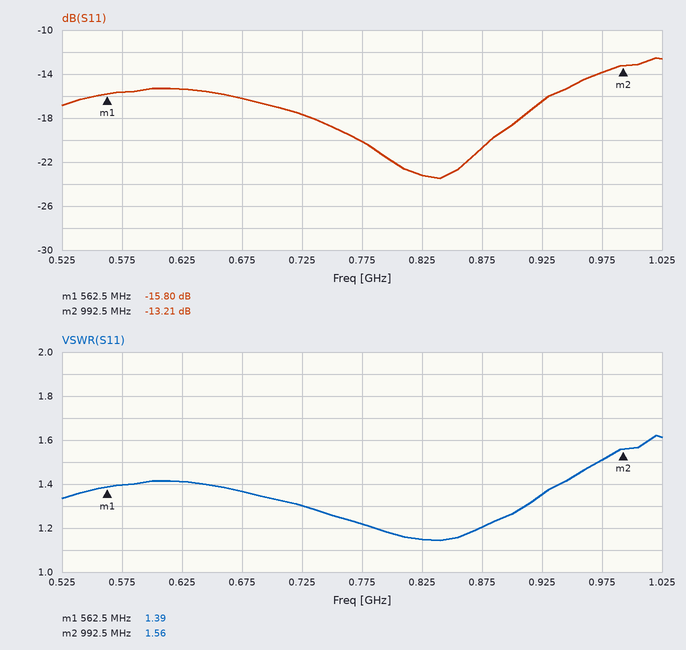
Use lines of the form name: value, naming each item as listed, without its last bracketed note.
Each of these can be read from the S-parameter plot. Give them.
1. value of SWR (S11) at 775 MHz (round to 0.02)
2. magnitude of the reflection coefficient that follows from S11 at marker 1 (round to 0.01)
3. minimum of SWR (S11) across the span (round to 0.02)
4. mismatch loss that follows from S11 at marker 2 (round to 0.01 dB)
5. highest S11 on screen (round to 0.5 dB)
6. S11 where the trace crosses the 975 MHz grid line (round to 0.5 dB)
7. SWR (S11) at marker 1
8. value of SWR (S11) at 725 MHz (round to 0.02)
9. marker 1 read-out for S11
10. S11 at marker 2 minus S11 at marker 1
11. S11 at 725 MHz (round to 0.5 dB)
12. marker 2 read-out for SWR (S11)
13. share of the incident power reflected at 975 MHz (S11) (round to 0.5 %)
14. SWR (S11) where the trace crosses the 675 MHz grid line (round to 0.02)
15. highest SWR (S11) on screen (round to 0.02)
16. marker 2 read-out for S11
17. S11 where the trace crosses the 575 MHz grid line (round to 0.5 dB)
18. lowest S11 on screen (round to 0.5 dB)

value of SWR (S11) at 775 MHz: 1.22
magnitude of the reflection coefficient that follows from S11 at marker 1: 0.16
minimum of SWR (S11) across the span: 1.14
mismatch loss that follows from S11 at marker 2: 0.21 dB
highest S11 on screen: -12.5 dB
S11 where the trace crosses the 975 MHz grid line: -14.0 dB
SWR (S11) at marker 1: 1.39
value of SWR (S11) at 725 MHz: 1.30
marker 1 read-out for S11: -15.80 dB
S11 at marker 2 minus S11 at marker 1: 2.59 dB
S11 at 725 MHz: -17.5 dB
marker 2 read-out for SWR: 1.56
share of the incident power reflected at 975 MHz (S11): 4.0 %
SWR (S11) where the trace crosses the 675 MHz grid line: 1.36
highest SWR (S11) on screen: 1.62
marker 2 read-out for S11: -13.21 dB
S11 where the trace crosses the 575 MHz grid line: -15.5 dB
lowest S11 on screen: -23.5 dB
